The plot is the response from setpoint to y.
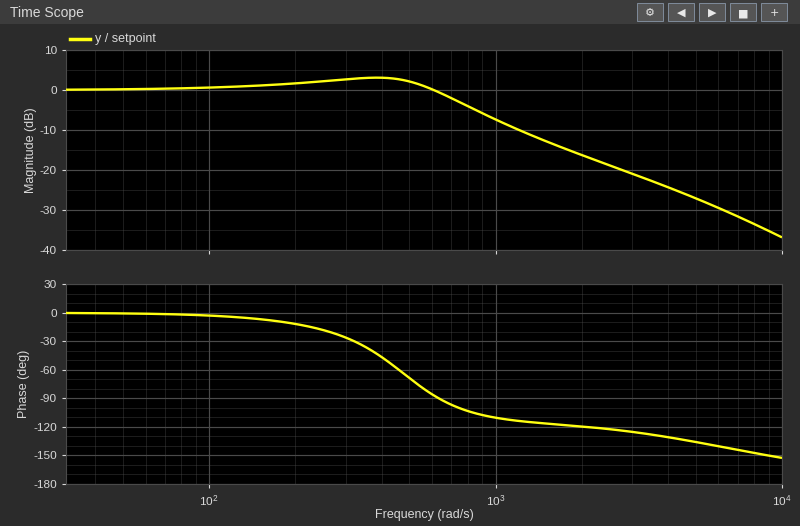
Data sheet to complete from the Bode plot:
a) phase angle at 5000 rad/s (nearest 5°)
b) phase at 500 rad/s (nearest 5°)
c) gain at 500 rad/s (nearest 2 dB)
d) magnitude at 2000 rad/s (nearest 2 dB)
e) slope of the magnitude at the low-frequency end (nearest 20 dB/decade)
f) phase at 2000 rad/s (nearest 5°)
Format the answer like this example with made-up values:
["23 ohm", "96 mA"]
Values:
["-135°", "-70°", "2 dB", "-16 dB", "0 dB/decade", "-120°"]
